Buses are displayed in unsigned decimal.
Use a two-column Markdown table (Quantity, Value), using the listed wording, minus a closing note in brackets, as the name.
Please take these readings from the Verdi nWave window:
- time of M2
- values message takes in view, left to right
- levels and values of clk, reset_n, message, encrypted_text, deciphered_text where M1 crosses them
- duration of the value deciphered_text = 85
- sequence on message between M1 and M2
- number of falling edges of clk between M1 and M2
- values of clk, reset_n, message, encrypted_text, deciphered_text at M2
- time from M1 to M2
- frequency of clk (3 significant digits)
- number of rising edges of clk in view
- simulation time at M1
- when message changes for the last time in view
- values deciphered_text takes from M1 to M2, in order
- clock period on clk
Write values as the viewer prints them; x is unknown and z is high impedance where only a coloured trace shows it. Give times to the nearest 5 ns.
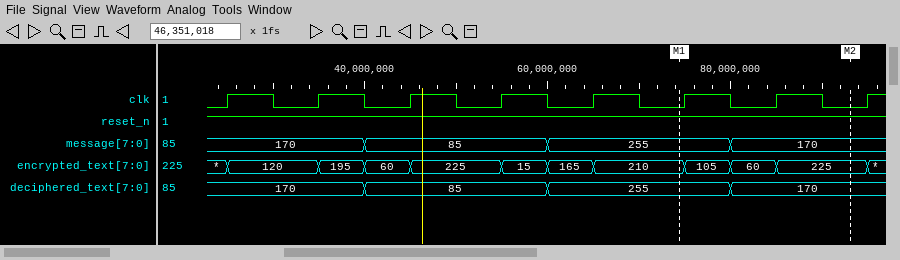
| Quantity | Value |
|---|---|
| time of M2 | 95 ns |
| values message takes in view, left to right | 170, 85, 255, 170 |
| levels and values of clk, reset_n, message, encrypted_text, deciphered_text where M1 crosses them | clk=0, reset_n=1, message=255, encrypted_text=210, deciphered_text=255 |
| duration of the value deciphered_text = 85 | 20 ns |
| sequence on message between M1 and M2 | 255, 170 |
| number of falling edges of clk between M1 and M2 | 2 |
| values of clk, reset_n, message, encrypted_text, deciphered_text at M2 | clk=0, reset_n=1, message=170, encrypted_text=225, deciphered_text=170 |
| time from M1 to M2 | 20 ns |
| frequency of clk | 100 MHz |
| number of rising edges of clk in view | 8 |
| simulation time at M1 | 75 ns |
| when message changes for the last time in view | 80 ns |
| values deciphered_text takes from M1 to M2, in order | 255, 170 |
| clock period on clk | 10 ns |
